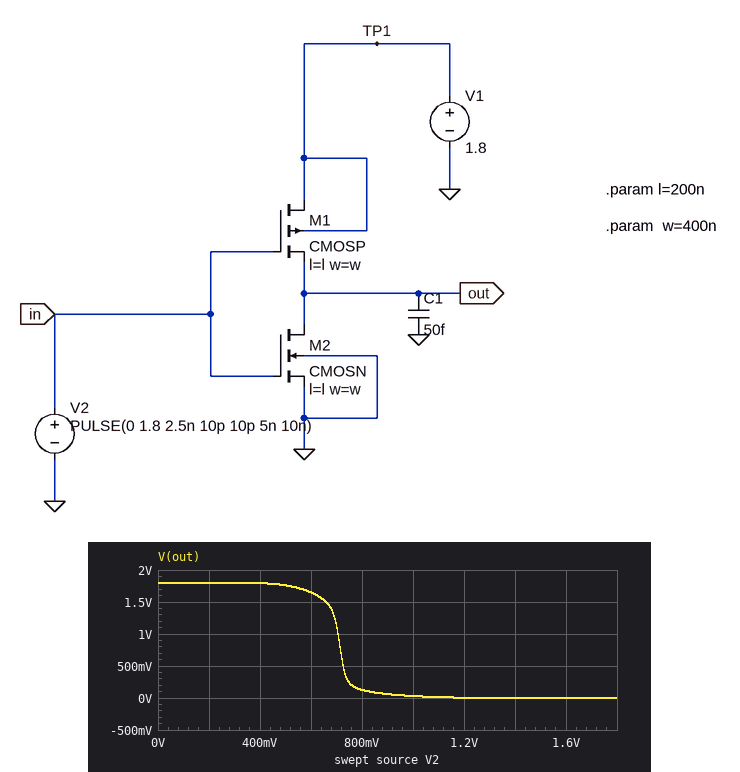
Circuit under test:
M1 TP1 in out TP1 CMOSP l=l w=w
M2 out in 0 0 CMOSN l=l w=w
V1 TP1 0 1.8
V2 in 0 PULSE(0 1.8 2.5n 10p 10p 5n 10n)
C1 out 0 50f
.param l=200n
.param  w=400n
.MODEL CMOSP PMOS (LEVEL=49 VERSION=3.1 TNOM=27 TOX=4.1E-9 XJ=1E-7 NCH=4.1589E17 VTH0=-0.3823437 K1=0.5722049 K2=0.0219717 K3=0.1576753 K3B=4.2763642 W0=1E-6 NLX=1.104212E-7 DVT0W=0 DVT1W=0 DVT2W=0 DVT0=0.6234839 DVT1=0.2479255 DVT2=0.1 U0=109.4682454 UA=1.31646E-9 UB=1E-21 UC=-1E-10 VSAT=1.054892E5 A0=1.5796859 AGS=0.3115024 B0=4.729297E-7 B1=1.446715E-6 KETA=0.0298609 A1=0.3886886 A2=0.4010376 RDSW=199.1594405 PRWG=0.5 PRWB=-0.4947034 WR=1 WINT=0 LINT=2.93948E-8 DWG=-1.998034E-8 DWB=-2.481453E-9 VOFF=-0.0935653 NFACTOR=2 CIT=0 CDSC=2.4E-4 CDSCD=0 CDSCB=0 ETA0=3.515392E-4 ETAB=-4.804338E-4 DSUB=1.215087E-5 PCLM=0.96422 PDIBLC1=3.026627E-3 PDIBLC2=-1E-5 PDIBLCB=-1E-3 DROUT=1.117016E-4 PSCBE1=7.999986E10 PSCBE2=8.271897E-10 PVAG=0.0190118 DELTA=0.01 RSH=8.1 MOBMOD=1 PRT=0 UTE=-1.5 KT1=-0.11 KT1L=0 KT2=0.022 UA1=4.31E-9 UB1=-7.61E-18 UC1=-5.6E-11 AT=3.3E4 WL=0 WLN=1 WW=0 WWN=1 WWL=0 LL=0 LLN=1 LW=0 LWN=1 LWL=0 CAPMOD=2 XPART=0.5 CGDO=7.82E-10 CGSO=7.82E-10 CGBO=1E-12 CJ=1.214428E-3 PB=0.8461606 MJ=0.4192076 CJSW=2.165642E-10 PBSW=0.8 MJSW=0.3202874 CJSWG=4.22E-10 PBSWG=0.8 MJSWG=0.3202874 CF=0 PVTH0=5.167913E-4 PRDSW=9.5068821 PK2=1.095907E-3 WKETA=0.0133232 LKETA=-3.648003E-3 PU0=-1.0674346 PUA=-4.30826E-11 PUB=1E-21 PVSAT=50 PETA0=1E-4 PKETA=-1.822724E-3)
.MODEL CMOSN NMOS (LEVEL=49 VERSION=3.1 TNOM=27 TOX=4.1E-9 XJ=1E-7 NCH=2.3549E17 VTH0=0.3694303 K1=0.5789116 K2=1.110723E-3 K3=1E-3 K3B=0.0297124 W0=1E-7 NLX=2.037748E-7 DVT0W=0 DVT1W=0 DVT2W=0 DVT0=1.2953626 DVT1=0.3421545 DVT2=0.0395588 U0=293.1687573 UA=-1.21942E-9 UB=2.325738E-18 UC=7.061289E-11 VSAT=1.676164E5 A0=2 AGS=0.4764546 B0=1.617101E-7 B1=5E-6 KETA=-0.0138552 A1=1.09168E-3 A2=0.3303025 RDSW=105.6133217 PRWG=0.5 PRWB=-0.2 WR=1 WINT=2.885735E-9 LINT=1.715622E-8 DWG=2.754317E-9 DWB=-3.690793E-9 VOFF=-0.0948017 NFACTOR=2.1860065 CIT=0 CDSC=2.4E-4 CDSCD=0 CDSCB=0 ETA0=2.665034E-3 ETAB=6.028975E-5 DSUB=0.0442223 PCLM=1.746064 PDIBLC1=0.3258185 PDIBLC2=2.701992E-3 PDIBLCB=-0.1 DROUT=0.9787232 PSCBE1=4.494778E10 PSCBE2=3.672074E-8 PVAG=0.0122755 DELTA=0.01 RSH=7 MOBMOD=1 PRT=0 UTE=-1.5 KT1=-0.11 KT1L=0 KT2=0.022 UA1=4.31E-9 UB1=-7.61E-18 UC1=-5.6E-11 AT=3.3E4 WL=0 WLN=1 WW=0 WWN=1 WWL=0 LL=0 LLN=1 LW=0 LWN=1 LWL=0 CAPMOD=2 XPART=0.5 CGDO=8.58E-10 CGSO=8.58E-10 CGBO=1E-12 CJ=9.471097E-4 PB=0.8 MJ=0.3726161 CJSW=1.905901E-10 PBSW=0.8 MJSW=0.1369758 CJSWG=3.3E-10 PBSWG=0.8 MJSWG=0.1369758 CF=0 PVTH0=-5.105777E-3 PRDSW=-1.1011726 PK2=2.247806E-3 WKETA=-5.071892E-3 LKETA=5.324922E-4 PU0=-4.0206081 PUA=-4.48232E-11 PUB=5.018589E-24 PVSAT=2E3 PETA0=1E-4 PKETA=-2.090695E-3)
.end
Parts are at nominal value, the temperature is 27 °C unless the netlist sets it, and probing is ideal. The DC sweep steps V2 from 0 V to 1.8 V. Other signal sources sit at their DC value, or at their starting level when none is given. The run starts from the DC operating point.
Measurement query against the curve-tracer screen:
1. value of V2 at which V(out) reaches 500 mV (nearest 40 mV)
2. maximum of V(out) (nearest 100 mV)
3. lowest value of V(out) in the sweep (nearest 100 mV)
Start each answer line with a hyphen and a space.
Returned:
- 720 mV
- 1.8 V
- 0 V
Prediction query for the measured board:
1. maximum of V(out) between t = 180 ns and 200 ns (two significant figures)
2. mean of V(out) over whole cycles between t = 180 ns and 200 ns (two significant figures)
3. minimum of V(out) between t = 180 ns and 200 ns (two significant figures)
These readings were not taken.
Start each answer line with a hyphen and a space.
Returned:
- 1.8 V
- 840 mV
- -28 mV
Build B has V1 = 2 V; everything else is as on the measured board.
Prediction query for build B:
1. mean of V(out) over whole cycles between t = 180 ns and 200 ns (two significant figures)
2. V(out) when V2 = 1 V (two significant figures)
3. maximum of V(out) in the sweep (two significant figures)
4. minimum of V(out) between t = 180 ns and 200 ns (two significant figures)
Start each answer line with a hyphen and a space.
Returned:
- 940 mV
- 73 mV
- 2.0 V
- -26 mV
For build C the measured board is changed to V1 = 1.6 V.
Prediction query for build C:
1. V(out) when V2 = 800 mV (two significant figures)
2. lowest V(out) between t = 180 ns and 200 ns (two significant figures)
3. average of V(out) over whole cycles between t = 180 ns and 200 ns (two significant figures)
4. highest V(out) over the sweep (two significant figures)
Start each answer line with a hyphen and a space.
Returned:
- 48 mV
- -29 mV
- 730 mV
- 1.6 V
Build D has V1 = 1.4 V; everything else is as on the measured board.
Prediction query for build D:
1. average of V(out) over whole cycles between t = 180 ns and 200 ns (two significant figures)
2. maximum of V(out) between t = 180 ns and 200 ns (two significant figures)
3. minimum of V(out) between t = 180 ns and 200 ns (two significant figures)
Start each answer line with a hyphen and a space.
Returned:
- 620 mV
- 1.4 V
- -30 mV
